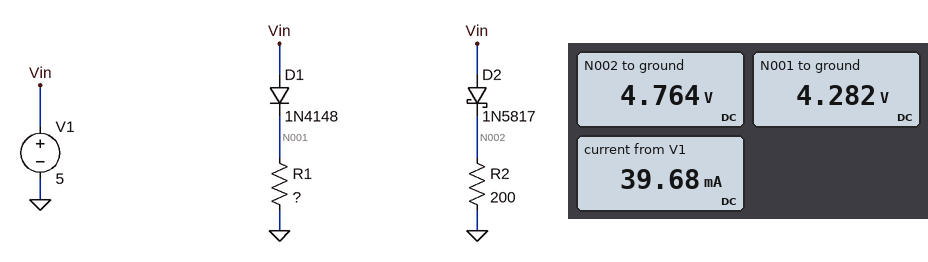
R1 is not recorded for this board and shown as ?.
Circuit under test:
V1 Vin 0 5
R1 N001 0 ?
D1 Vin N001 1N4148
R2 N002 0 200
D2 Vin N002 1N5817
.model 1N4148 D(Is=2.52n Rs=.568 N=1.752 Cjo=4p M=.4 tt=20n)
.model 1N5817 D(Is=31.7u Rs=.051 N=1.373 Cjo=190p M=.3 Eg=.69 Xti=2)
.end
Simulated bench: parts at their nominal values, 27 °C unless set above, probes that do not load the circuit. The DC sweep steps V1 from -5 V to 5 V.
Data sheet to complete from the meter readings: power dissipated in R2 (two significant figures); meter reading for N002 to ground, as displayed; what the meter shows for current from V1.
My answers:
110 mW
4.764 V
39.68 mA
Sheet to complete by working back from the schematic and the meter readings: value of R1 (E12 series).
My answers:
270 Ω
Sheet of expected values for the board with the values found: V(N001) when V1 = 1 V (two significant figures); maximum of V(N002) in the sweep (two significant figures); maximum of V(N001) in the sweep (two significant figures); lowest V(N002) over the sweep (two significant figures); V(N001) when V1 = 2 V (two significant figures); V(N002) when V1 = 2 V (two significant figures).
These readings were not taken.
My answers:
400 mV
4.8 V
4.3 V
-6.3 mV
1.3 V
1.8 V
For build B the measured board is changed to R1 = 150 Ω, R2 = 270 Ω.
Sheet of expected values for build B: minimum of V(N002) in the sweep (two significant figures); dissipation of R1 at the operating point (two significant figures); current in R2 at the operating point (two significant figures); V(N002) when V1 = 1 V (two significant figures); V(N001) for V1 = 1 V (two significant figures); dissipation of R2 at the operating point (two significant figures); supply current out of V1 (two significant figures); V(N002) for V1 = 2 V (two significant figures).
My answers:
-8.6 mV
120 mW
18 mA
840 mV
370 mV
84 mW
46 mA
1.8 V
